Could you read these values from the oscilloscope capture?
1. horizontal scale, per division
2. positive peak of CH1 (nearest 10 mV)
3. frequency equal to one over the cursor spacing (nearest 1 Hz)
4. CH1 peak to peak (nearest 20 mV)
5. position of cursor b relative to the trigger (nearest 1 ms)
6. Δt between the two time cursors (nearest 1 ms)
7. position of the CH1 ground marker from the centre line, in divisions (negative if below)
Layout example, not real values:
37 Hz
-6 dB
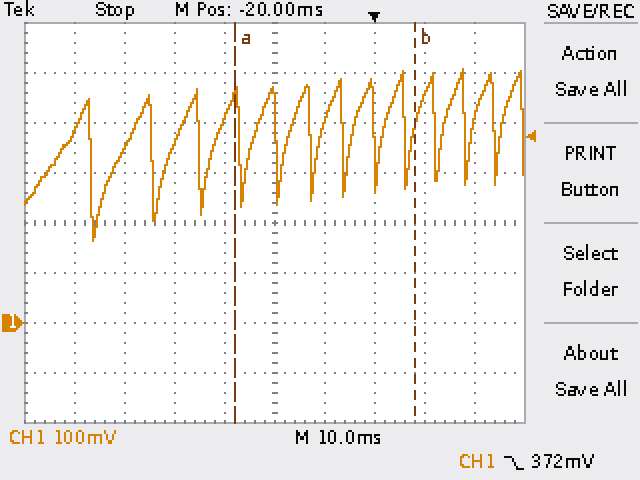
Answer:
10 ms
510 mV
28 Hz
340 mV
+8 ms
36 ms
-2.0 div
